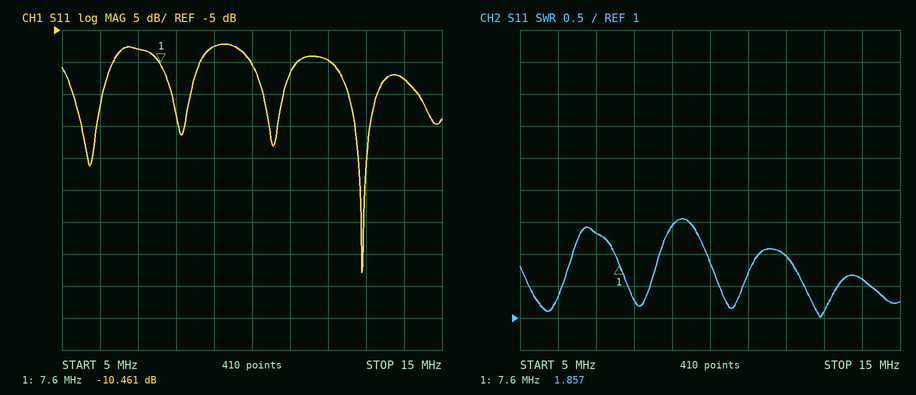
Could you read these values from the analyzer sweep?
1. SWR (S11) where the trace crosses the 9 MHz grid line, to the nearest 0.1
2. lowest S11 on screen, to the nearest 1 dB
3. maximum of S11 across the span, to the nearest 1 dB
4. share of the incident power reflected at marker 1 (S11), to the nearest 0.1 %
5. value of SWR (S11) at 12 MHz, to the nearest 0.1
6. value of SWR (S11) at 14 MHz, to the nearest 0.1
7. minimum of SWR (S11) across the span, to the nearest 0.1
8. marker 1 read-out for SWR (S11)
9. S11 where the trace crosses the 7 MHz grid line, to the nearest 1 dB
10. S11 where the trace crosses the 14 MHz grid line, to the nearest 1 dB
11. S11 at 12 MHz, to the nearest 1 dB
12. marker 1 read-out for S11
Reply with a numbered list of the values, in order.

1. 2.4
2. -43 dB
3. -7 dB
4. 9.0 %
5. 2.0
6. 1.6
7. 1.0
8. 1.857
9. -8 dB
10. -13 dB
11. -10 dB
12. -10.461 dB
